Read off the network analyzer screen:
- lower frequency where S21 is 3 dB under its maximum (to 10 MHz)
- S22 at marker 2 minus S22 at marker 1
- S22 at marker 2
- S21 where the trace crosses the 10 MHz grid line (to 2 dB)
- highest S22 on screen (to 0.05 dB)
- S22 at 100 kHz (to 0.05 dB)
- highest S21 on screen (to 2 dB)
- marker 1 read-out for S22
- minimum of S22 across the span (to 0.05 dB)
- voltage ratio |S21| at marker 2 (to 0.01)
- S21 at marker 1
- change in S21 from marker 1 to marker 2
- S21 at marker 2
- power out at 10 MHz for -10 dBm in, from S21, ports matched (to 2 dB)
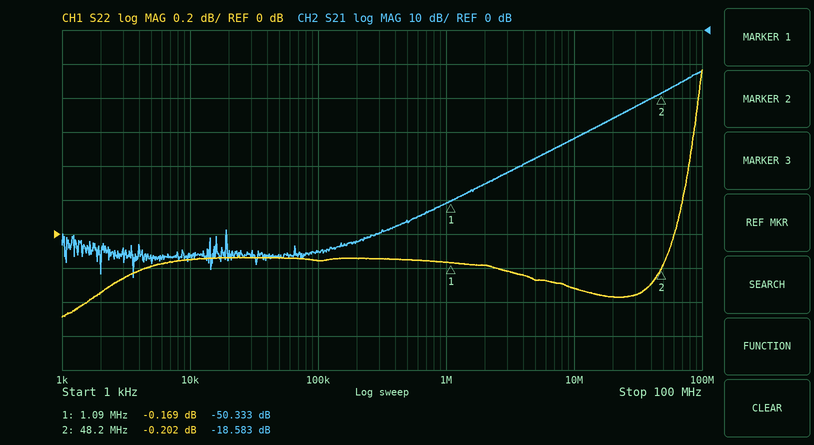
70 MHz
-0.033 dB
-0.202 dB
-32 dB
0.95 dB
-0.15 dB
-12 dB
-0.169 dB
-0.50 dB
0.12
-50.333 dB
31.750 dB
-18.583 dB
-42 dBm
